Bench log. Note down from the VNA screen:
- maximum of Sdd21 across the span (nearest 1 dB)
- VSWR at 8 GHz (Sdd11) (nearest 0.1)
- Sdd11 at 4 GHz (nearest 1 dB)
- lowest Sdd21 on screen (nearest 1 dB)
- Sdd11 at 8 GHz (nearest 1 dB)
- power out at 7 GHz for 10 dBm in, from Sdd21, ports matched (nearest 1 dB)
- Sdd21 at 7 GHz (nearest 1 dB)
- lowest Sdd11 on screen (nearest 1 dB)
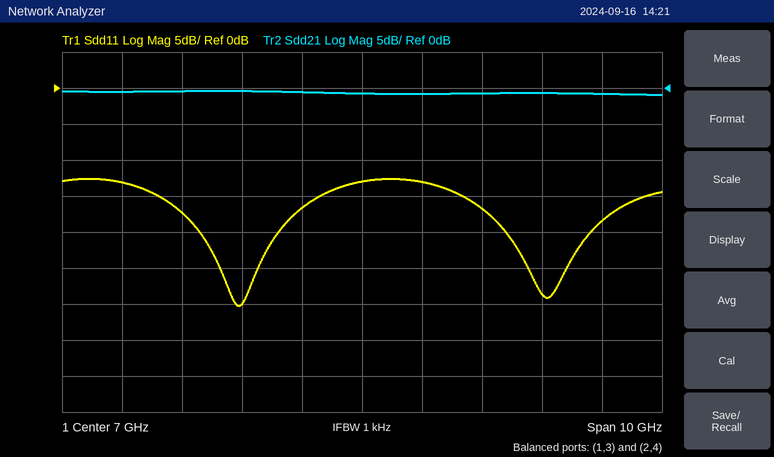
0 dB
1.6
-17 dB
-1 dB
-13 dB
9 dBm
-1 dB
-30 dB
